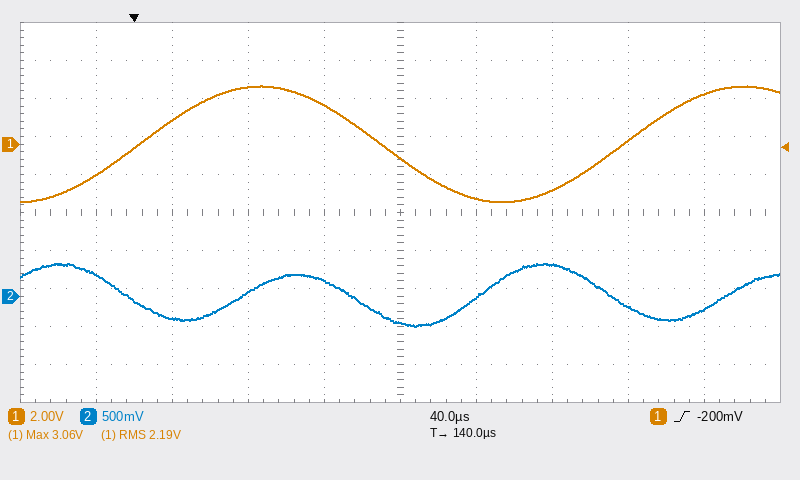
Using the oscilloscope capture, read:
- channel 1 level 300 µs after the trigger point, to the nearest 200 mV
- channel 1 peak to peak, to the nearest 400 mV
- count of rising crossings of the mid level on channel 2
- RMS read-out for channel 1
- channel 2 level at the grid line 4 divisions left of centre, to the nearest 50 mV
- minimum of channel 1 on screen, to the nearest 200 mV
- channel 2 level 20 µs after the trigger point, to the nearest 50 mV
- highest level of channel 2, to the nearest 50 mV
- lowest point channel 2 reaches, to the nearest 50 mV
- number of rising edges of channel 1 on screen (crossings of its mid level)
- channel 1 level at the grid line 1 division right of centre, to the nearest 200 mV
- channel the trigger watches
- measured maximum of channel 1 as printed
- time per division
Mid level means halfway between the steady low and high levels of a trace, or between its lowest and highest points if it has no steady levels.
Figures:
2.6 V
6.0 V
3
2.19 V
300 mV
-3.0 V
-300 mV
450 mV
-400 mV
2
-2.8 V
channel 1
3.06 V
40 µs
